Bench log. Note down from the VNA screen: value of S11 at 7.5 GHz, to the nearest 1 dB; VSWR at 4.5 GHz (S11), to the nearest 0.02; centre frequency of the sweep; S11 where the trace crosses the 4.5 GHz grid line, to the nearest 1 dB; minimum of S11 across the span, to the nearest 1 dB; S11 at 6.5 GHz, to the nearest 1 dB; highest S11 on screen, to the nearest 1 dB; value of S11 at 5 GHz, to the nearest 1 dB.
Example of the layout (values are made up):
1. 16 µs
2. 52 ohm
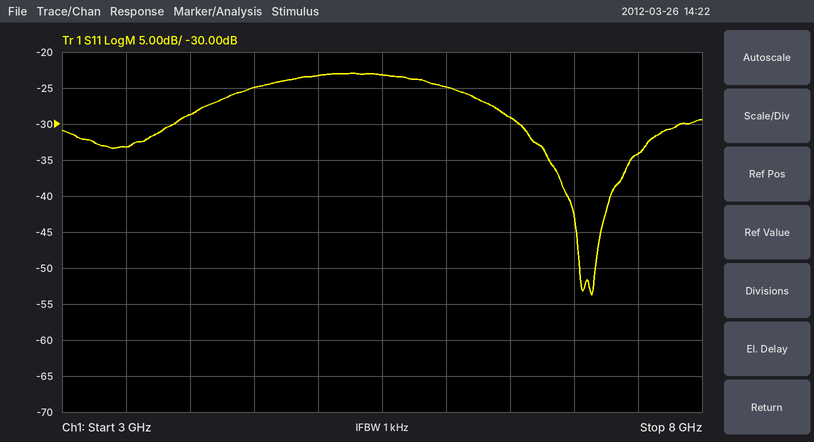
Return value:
1. -34 dB
2. 1.12
3. 5.5 GHz
4. -25 dB
5. -54 dB
6. -29 dB
7. -23 dB
8. -23 dB
